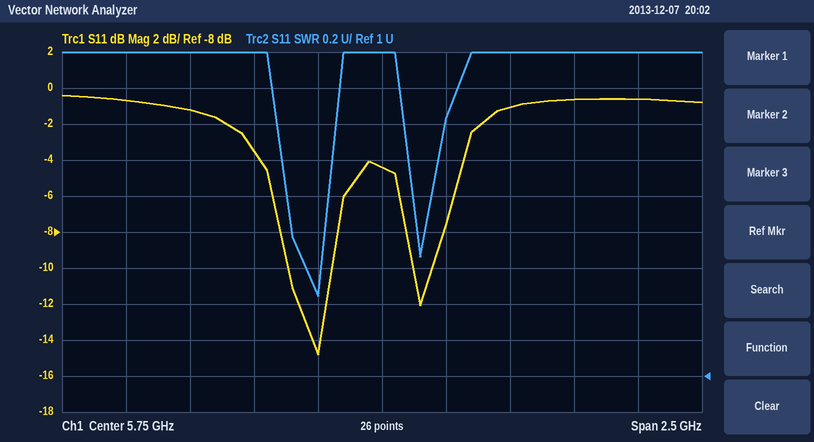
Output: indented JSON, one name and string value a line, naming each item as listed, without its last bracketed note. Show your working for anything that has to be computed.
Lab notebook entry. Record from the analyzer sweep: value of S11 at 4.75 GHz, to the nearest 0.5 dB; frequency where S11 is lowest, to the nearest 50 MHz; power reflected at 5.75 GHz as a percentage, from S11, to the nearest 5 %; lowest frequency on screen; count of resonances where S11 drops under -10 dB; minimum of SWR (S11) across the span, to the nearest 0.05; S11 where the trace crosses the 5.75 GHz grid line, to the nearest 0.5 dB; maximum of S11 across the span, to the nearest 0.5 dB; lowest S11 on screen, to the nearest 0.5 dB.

{
  "value of S11 at 4.75 GHz, to the nearest 0.5 dB": "-0.5 dB",
  "frequency where S11 is lowest, to the nearest 50 MHz": "5.50 GHz",
  "power reflected at 5.75 GHz as a percentage, from S11, to the nearest 5 %": "10^(-4.5/10) ≈ 35 %",
  "lowest frequency on screen": "4.5 GHz",
  "count of resonances where S11 drops under -10 dB": "2",
  "minimum of SWR (S11) across the span, to the nearest 0.05": "1.45",
  "S11 where the trace crosses the 5.75 GHz grid line, to the nearest 0.5 dB": "-4.5 dB",
  "maximum of S11 across the span, to the nearest 0.5 dB": "-0.5 dB",
  "lowest S11 on screen, to the nearest 0.5 dB": "-15.0 dB"
}
